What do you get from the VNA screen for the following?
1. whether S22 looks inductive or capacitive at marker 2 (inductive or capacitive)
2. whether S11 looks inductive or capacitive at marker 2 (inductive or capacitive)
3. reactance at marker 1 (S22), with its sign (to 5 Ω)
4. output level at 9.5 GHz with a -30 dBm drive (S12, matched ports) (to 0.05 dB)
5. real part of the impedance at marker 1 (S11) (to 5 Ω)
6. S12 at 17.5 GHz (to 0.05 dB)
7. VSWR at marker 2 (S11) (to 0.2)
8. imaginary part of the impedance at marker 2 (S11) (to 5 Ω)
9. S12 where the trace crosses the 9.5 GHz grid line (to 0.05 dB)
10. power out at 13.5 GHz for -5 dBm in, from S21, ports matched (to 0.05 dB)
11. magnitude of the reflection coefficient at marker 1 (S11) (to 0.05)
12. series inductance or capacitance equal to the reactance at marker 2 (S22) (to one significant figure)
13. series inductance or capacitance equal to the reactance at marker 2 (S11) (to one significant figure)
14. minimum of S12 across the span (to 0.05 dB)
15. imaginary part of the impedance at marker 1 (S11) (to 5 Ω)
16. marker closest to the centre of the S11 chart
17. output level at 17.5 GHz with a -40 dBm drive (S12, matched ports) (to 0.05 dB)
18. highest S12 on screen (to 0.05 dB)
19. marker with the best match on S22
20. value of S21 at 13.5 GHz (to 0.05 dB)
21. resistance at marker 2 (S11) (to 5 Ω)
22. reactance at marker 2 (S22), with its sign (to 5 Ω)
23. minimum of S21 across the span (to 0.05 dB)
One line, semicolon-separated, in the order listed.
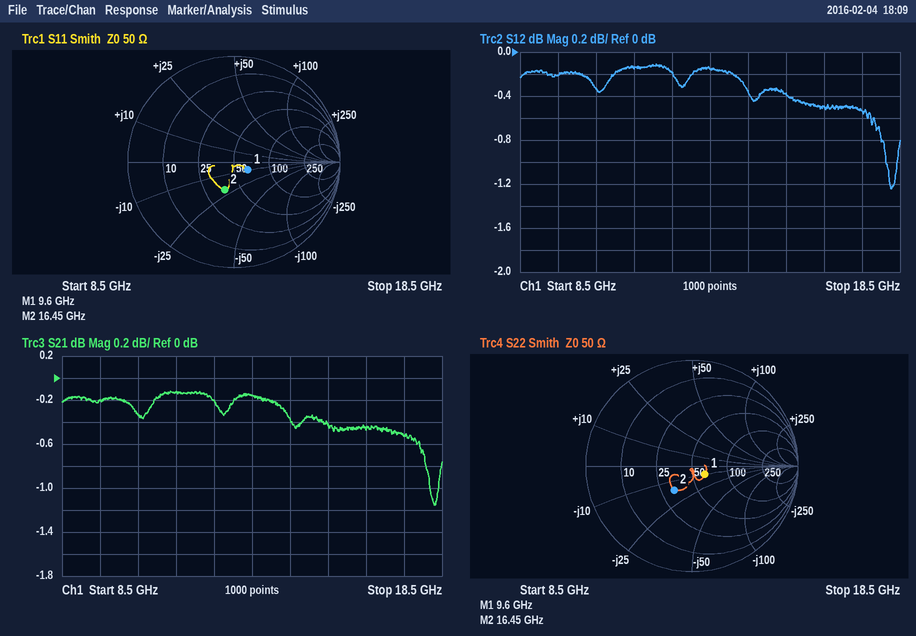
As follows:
capacitive; capacitive; -10 Ω; -30.20 dBm; 65 Ω; -0.55 dB; 1.8; -20 Ω; -0.20 dB; -5.15 dBm; 0.15; 600 fF; 500 fF; -1.25 dB; -10 Ω; marker 1; -40.55 dBm; -0.10 dB; marker 1; -0.15 dB; 35 Ω; -15 Ω; -1.15 dB
